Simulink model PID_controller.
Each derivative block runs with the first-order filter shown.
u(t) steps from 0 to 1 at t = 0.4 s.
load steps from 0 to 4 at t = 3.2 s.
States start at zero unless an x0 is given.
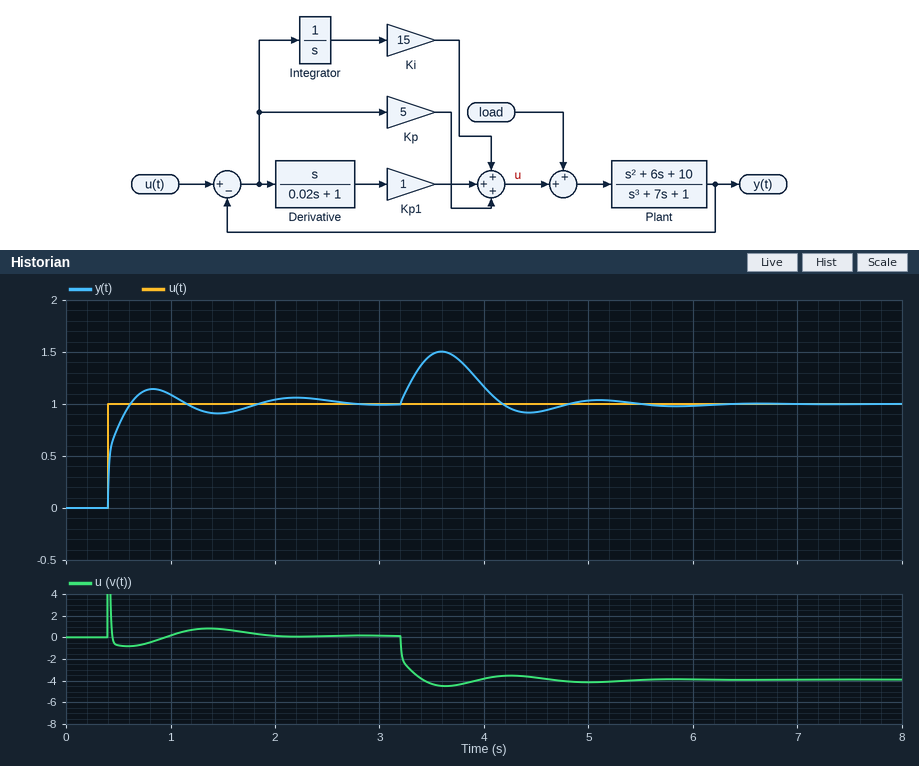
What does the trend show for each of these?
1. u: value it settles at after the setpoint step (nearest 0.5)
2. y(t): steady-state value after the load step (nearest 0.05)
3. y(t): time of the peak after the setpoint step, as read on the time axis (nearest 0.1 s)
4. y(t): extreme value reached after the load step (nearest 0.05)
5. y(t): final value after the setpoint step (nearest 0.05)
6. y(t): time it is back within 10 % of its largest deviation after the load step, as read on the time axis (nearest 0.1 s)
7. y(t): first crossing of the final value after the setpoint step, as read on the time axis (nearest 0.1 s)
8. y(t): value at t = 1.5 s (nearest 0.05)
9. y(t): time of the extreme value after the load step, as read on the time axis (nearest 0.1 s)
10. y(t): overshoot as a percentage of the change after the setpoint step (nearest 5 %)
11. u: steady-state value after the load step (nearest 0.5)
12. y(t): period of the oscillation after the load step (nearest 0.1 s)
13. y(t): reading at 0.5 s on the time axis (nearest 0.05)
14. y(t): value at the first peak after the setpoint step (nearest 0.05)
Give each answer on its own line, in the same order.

0.0
1.00
0.8 s
1.50
1.00
4.6 s
0.6 s
0.90
3.6 s
15 %
-4.0
1.5 s
0.80
1.15
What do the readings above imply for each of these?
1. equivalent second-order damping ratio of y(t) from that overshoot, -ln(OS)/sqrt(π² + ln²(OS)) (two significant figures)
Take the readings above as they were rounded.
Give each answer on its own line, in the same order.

0.52
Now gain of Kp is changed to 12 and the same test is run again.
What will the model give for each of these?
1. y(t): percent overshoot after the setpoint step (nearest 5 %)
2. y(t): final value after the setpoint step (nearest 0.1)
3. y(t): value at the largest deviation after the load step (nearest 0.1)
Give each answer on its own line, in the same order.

10 %
1.0
1.3
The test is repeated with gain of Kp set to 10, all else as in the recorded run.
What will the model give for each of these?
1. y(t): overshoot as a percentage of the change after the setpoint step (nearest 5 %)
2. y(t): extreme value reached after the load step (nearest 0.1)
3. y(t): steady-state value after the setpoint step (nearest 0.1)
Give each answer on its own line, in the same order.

10 %
1.3
1.0
